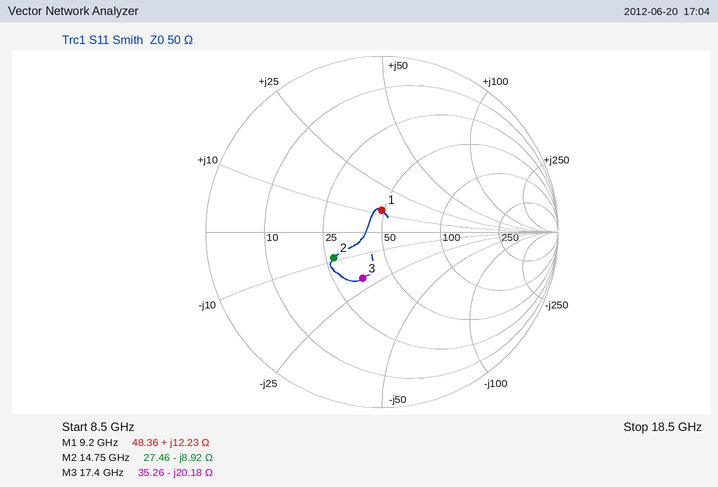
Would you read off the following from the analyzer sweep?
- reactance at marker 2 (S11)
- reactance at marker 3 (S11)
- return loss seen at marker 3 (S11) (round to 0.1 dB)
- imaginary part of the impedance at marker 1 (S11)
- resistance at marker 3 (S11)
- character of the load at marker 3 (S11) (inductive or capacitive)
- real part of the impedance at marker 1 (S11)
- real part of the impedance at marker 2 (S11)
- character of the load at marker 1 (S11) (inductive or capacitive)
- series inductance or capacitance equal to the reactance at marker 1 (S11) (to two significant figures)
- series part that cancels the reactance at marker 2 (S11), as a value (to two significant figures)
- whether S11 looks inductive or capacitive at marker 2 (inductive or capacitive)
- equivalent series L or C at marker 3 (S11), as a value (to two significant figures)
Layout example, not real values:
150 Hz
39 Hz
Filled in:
-8.92 Ω
-20.18 Ω
10.9 dB
+12.23 Ω
35.26 Ω
capacitive
48.36 Ω
27.46 Ω
inductive
210 pH
96 pH
capacitive
450 fF
